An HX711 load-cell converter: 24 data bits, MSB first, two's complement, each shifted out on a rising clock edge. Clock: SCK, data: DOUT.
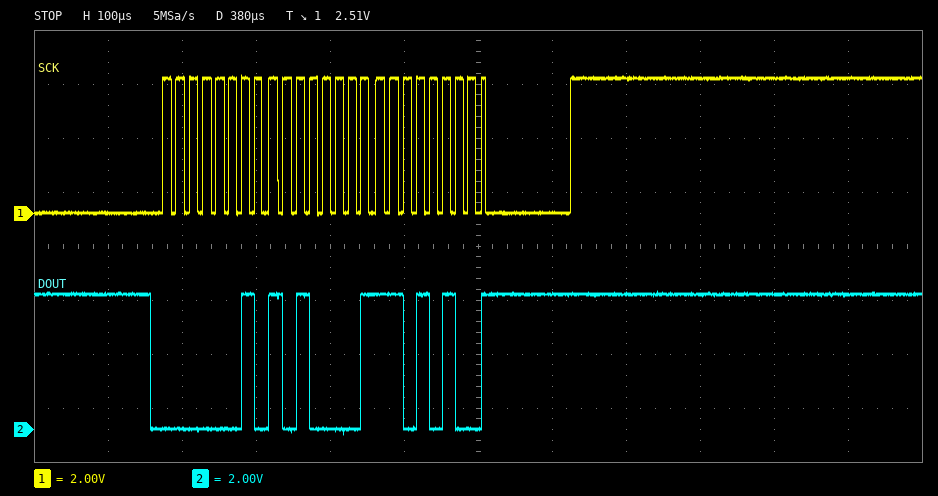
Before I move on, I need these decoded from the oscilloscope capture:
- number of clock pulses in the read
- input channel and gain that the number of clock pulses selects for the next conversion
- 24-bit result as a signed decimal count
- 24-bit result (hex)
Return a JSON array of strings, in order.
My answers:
["26", "channel B, gain 32", "172500", "0x02A1D4"]
